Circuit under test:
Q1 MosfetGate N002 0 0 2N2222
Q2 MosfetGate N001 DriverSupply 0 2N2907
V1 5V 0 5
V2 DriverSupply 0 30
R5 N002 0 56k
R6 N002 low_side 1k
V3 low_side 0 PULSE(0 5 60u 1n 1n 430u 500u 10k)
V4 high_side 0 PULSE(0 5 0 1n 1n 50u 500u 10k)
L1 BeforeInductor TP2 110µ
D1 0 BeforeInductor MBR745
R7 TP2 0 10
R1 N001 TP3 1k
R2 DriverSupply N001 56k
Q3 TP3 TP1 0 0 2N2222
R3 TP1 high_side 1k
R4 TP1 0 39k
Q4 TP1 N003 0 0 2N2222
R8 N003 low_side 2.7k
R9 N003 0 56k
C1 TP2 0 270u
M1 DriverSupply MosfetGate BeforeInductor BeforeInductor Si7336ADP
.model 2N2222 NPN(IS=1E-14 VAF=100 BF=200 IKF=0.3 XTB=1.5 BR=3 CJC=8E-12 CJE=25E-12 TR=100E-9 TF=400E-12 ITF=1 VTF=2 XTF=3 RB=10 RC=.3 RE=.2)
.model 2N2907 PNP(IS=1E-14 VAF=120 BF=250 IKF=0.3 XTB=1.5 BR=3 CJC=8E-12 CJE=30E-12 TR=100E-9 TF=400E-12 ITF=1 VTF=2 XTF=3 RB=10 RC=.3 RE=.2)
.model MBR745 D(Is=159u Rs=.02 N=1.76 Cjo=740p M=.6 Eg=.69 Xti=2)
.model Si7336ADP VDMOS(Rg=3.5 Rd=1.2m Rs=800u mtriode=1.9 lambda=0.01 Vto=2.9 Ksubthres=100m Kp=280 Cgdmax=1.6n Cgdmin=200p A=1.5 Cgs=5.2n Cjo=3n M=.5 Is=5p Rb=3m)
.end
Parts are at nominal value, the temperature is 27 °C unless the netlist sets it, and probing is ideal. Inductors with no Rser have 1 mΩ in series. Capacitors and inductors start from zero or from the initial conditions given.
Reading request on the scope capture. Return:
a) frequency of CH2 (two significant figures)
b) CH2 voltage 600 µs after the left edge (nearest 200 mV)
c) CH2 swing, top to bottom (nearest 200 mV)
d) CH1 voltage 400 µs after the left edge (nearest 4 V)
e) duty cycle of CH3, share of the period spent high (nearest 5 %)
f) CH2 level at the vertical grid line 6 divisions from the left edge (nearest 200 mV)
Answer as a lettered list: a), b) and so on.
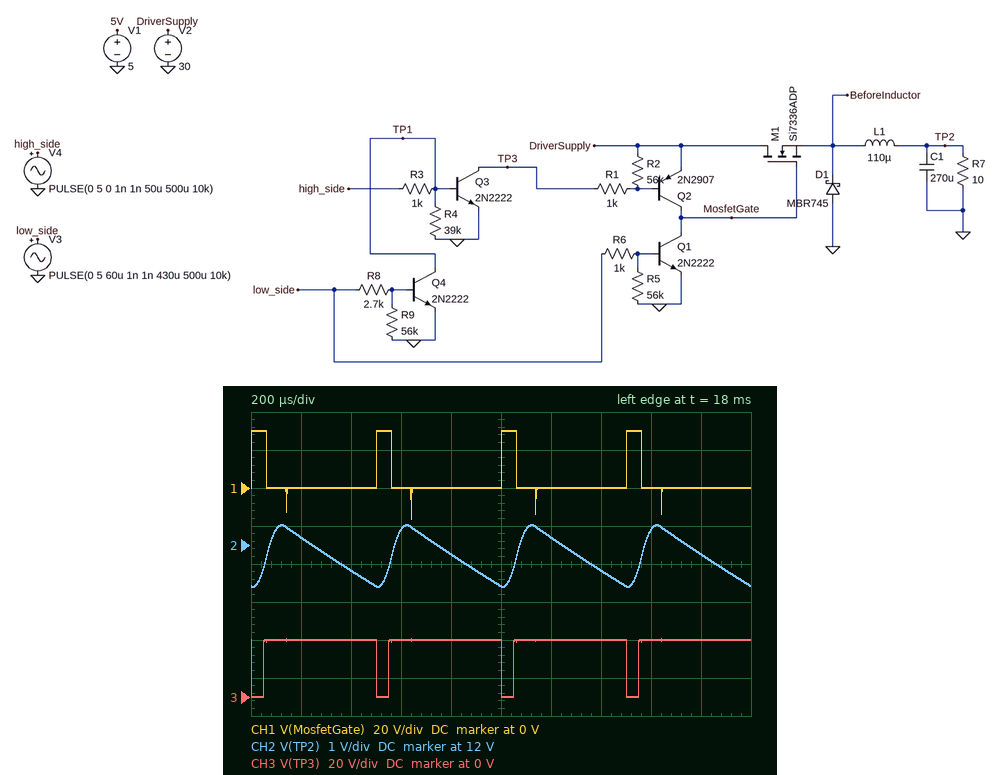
a) 2.0 kHz
b) 12.4 V
c) 1.6 V
d) 0 V
e) 90 %
f) 12.2 V
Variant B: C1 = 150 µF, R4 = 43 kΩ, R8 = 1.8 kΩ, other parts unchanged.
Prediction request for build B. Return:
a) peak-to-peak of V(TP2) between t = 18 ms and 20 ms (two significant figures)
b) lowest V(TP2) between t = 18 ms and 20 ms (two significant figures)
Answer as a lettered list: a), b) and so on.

a) 3.0 V
b) 10 V
